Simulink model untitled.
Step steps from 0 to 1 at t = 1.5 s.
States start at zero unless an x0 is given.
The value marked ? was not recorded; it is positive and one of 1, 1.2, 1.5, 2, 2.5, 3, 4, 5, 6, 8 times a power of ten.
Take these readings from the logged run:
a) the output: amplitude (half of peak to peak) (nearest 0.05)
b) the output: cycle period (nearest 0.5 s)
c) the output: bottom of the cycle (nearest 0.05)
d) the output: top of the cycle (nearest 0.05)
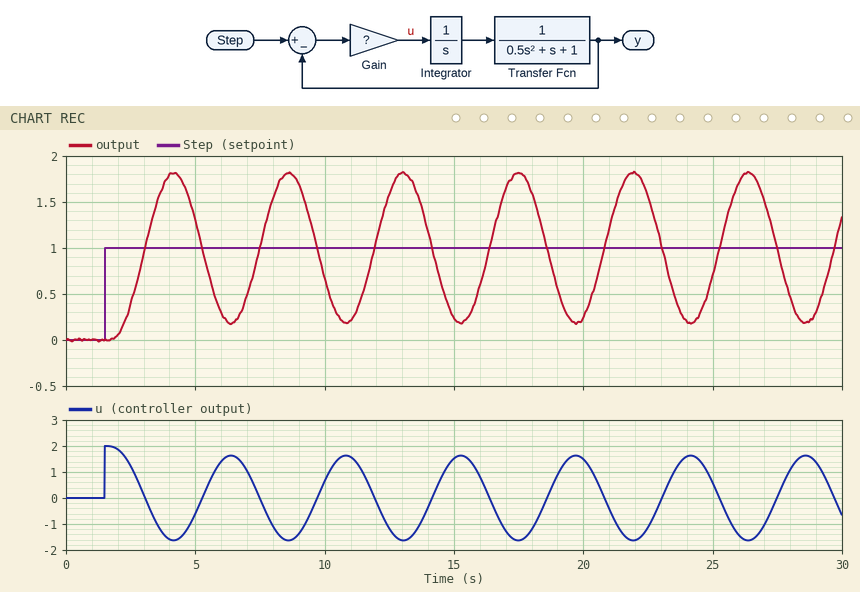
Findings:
0.80
4.5 s
0.20
1.80
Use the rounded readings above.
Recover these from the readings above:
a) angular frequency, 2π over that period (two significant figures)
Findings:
1.4 rad/s
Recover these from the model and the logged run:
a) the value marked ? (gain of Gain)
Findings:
2
